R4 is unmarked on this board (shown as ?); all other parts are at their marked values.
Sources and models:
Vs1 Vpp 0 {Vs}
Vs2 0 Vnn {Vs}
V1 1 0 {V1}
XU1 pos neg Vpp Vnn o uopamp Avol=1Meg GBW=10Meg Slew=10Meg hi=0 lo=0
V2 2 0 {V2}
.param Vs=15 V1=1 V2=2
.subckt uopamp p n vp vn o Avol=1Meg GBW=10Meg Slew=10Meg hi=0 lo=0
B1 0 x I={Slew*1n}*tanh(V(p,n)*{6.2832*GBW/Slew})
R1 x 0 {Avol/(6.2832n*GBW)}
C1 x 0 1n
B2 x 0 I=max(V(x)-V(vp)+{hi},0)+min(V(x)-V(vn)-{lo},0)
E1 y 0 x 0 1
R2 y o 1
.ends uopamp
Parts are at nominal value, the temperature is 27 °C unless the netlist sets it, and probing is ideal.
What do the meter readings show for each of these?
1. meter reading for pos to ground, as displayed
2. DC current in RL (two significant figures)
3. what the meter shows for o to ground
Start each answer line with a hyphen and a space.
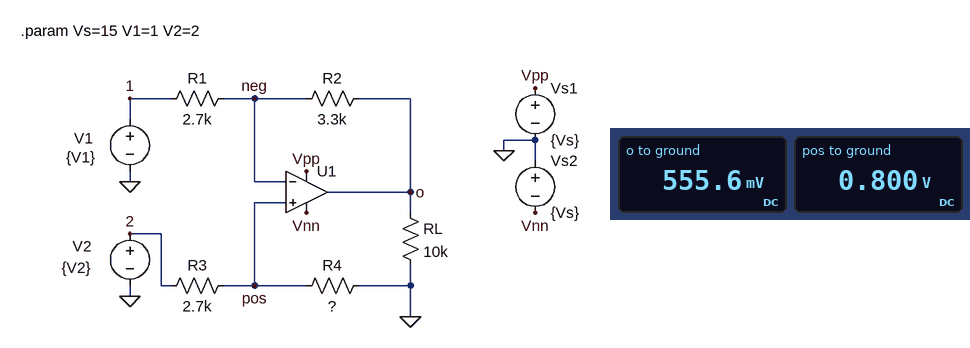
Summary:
- 0.800 V
- 56 µA
- 555.6 mV
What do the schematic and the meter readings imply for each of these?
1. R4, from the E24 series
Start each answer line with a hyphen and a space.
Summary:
- 1.8 kΩ
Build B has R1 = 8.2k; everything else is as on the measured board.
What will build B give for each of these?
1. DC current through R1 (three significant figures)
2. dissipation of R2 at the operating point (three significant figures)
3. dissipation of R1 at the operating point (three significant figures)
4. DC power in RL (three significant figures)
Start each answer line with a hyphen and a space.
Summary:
- 24.4 µA
- 1.96 µW
- 4.88 µW
- 51.8 µW
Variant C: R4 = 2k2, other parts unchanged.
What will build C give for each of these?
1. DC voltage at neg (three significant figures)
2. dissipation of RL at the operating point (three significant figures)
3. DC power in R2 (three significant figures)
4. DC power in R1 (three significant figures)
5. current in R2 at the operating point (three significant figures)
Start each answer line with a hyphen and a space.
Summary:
- 898 mV
- 59.8 µW
- 4.71 µW
- 3.86 µW
- 37.8 µA
